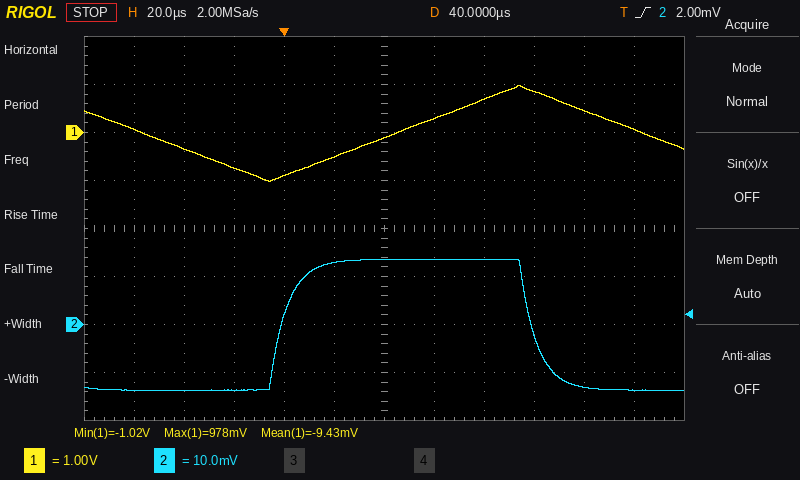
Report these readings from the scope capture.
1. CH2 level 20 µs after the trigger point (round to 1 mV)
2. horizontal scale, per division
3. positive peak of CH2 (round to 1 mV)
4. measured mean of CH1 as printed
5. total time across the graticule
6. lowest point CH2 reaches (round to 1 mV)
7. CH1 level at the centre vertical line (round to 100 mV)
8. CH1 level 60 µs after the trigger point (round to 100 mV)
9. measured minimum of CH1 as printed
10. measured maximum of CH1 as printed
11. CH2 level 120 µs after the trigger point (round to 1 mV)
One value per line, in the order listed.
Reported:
13 mV
20 µs
14 mV
-9.43 mV
240 µs
-14 mV
-100 mV
300 mV
-1.02 V
978 mV
-13 mV
